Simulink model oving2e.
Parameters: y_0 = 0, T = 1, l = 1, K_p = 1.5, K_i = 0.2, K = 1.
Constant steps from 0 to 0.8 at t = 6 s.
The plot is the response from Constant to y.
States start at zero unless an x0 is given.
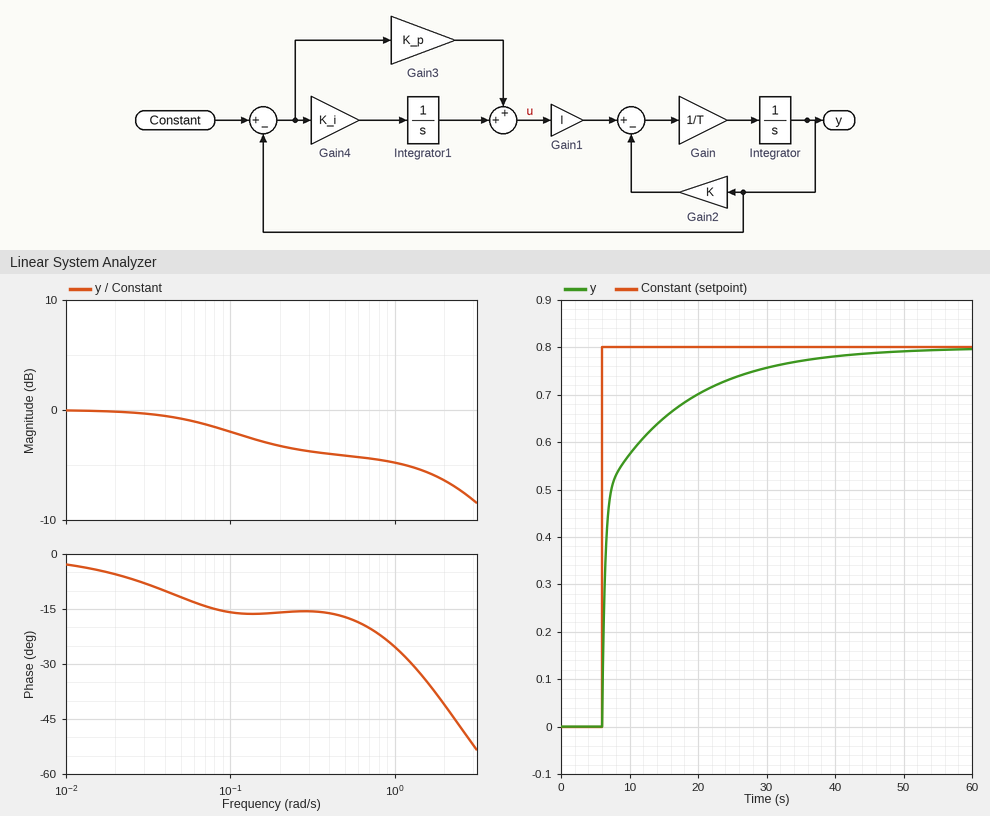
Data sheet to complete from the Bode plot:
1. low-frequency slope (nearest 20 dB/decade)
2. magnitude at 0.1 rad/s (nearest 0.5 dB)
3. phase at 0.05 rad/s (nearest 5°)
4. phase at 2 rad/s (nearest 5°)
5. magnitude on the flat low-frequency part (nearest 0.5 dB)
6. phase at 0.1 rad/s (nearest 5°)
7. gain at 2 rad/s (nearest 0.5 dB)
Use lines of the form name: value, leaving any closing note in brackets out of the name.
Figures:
low-frequency slope: 0 dB/decade
magnitude at 0.1 rad/s: -2.0 dB
phase at 0.05 rad/s: -10°
phase at 2 rad/s: -40°
magnitude on the flat low-frequency part: 0.0 dB
phase at 0.1 rad/s: -15°
gain at 2 rad/s: -6.5 dB
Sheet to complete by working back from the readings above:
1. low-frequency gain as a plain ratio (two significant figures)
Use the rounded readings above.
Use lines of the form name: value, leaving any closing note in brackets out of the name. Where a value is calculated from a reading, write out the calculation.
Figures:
low-frequency gain as a plain ratio: 10^(0 / 20) = 1.0
